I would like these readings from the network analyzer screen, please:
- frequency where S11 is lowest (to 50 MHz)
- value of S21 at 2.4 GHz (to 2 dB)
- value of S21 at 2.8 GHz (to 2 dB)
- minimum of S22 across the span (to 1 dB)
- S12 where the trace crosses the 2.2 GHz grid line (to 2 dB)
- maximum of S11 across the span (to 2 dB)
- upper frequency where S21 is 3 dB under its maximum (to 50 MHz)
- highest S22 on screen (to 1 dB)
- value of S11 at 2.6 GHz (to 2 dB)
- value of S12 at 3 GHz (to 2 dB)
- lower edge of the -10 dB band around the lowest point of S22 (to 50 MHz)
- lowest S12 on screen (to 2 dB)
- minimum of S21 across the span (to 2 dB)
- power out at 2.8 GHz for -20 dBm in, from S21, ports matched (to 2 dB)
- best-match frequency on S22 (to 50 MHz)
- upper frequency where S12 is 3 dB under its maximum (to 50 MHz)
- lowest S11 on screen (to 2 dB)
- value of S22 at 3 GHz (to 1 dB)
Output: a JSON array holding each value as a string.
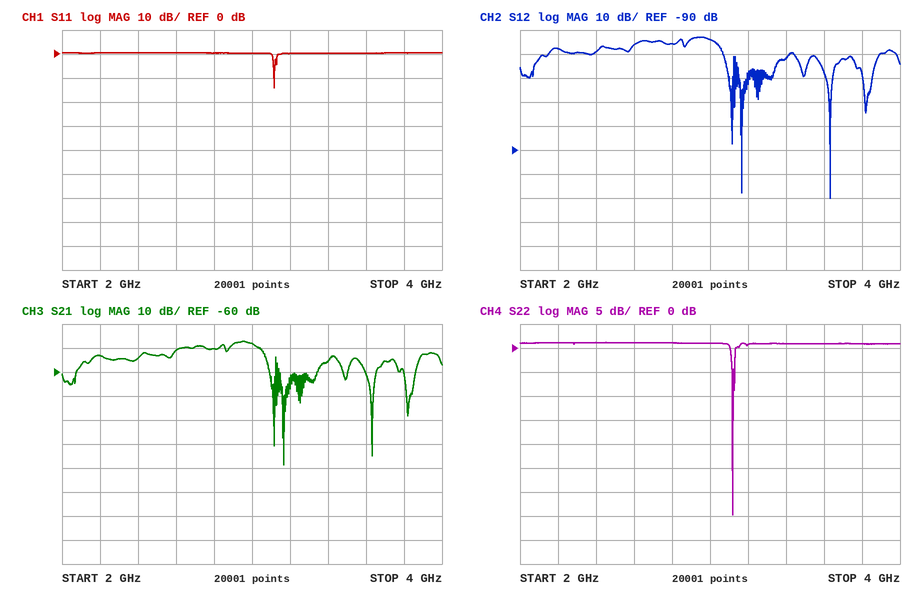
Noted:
["3.10 GHz", "-54 dB", "-50 dB", "-35 dB", "-48 dB", "0 dB", "3.05 GHz", "1 dB", "0 dB", "-44 dB", "3.10 GHz", "-110 dB", "-98 dB", "-70 dBm", "3.10 GHz", "3.05 GHz", "-14 dB", "1 dB"]
